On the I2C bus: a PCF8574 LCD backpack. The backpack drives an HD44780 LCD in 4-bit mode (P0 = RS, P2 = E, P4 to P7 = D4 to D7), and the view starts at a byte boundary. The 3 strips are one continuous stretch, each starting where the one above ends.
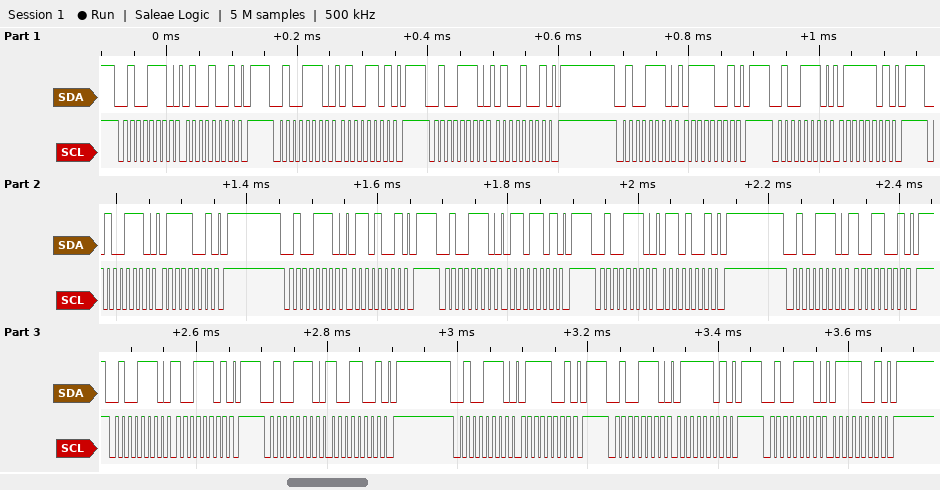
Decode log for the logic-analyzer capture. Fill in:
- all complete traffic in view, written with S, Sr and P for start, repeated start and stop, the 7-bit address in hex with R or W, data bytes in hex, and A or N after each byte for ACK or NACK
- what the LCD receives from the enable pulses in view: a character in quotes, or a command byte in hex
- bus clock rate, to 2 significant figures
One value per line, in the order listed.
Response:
S 27W A 49 A P S 27W A 4D A P S 27W A 49 A P S 27W A 79 A P S 27W A 7D A P S 27W A 79 A P S 27W A 69 A P S 27W A 6D A P S 27W A 69 A P S 27W A 99 A P S 27W A 9D A P S 27W A 99 A P S 27W A 79 A P S 27W A 7D A P S 27W A 79 A P
'G' 'i'
100 kHz
